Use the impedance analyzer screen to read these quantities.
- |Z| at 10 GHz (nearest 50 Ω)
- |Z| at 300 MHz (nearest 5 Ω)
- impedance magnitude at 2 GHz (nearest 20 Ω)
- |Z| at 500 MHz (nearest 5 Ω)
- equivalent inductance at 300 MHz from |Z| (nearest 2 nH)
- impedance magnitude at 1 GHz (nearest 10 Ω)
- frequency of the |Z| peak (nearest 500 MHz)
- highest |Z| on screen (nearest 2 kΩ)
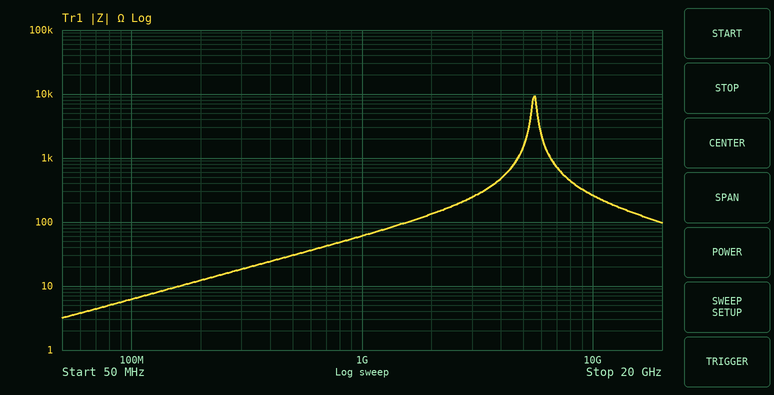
250 Ω
20 Ω
140 Ω
30 Ω
10 nH
60 Ω
5.5 GHz
10 kΩ
